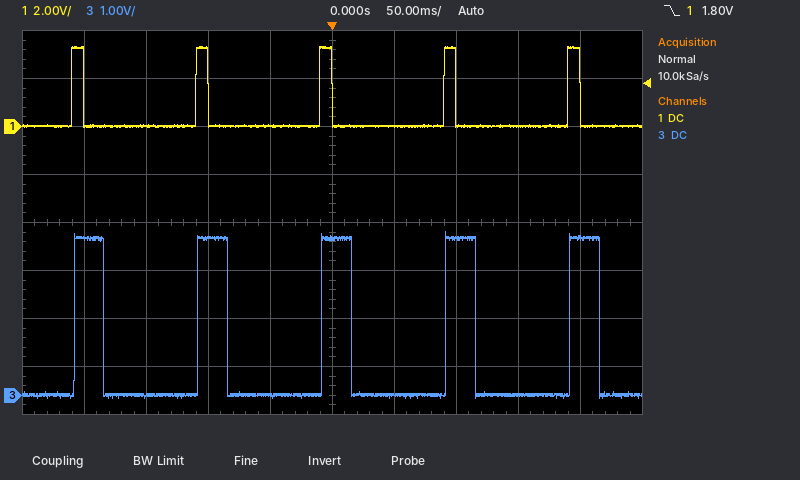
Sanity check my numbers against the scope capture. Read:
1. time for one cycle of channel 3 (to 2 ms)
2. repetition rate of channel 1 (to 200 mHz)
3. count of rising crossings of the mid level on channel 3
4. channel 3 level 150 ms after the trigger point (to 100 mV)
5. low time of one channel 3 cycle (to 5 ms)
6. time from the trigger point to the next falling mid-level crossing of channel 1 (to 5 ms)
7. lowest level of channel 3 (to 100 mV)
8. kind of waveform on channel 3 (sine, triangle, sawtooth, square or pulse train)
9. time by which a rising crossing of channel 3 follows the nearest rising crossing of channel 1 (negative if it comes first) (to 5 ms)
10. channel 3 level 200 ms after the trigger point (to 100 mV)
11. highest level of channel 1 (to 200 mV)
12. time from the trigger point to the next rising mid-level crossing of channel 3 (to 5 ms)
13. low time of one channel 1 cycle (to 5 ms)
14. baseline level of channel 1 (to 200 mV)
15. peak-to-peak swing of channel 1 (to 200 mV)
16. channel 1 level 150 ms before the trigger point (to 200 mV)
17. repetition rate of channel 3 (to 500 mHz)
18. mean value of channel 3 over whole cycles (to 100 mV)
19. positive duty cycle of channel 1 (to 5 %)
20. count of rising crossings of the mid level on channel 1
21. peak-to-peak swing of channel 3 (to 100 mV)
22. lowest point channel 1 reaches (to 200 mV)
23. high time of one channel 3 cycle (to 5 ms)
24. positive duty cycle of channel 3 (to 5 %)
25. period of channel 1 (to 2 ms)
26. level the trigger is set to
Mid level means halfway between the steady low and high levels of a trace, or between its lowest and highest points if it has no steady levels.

100 ms
10.0 Hz
5
0.0 V
75 ms
100 ms
-100 mV
pulse train
0 ms
3.3 V
3.4 V
90 ms
90 ms
0.0 V
3.4 V
0.0 V
10.0 Hz
800 mV
10 %
5
3.5 V
0.0 V
25 ms
25 %
100 ms
1.80 V
